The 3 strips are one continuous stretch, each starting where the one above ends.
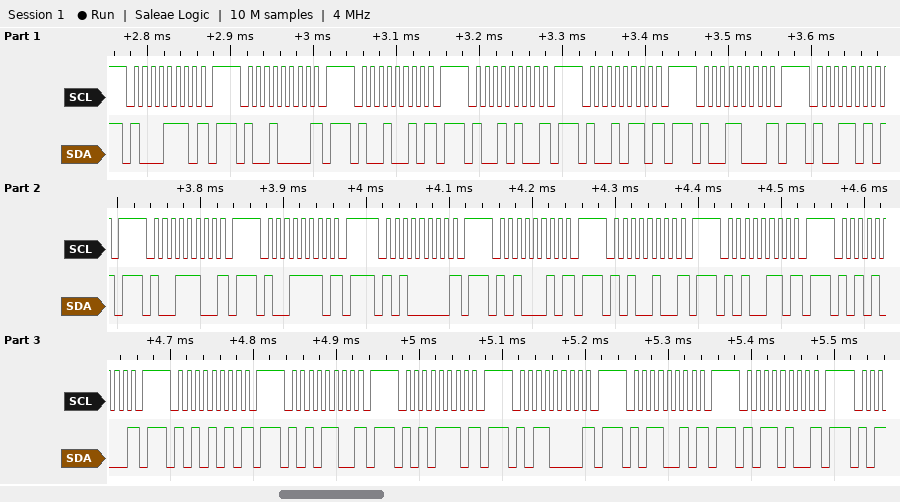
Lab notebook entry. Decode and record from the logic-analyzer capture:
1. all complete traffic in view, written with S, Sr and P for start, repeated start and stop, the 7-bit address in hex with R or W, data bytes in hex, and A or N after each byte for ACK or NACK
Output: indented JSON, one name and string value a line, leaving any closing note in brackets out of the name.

{
  "all complete traffic in view, written with S, Sr and P for start, repeated start and stop, the 7-bit address in hex with R or W, data bytes in hex, and A or N after each byte for ACK or NACK": "S 47W N P S 48W N P S 49W N P S 4AW N P S 4BW N P S 4CW N P S 4DW N P S 4EW N P S 4FW N P S 50W N P S 51W N P S 52W N P S 53W N P S 54W N P S 55W N P S 56W N P S 57W N P S 58W N P S 59W N P S 5AW N P"
}
